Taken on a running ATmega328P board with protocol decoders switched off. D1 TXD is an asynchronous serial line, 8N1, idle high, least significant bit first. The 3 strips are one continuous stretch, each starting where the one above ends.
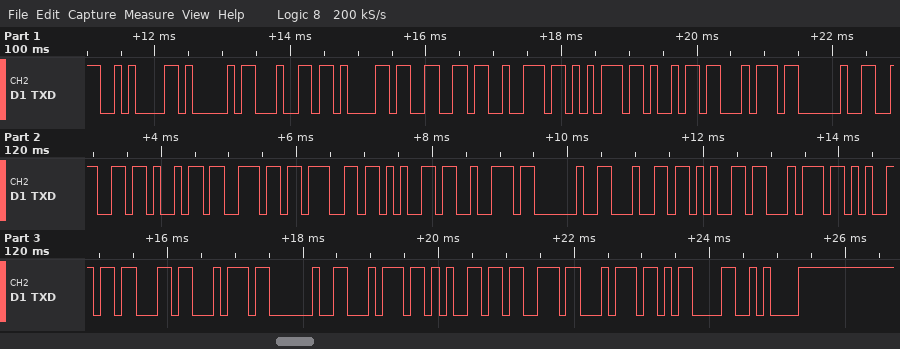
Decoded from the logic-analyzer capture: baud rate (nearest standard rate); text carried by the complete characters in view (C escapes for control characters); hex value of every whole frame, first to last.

9600 baud
"\nAdafruit finger detect test\r\n"
0A 41 64 61 66 72 75 69 74 20 66 69 6E 67 65 72 20 64 65 74 65 63 74 20 74 65 73 74 0D 0A
